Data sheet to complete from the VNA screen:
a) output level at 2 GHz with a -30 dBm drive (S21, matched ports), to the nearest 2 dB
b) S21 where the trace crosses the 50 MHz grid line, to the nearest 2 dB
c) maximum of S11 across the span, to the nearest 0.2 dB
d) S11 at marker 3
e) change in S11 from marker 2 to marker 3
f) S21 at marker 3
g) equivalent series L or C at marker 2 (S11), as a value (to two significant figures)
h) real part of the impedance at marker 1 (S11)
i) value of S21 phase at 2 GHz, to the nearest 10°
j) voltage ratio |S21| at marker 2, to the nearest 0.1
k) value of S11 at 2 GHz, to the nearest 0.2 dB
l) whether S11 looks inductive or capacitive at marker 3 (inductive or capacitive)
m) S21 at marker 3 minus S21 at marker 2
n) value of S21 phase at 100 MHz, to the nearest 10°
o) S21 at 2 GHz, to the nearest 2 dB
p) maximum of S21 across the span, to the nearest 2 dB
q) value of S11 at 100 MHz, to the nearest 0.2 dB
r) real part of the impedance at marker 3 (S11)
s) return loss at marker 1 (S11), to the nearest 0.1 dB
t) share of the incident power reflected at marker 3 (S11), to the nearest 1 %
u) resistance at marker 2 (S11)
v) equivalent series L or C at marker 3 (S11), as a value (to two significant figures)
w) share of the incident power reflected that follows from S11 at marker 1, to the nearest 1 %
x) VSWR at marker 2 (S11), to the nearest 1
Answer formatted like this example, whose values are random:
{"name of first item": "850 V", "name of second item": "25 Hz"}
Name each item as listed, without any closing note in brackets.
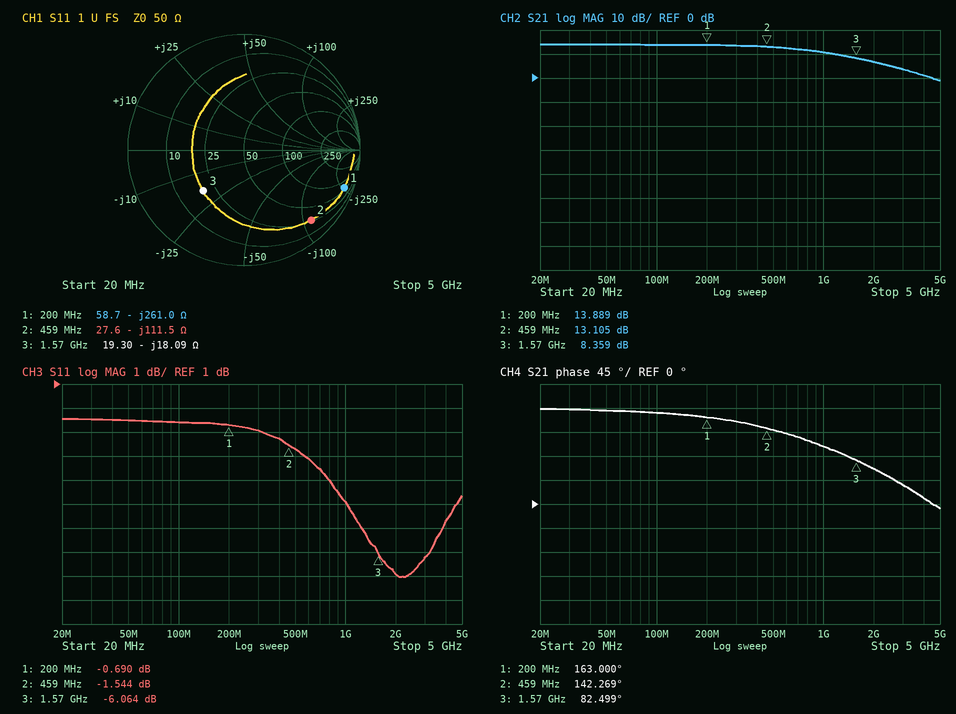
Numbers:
{"output level at 2 GHz with a -30 dBm drive (S21, matched ports), to the nearest 2 dB": "-24 dBm", "S21 where the trace crosses the 50 MHz grid line, to the nearest 2 dB": "14 dB", "maximum of S11 across the span, to the nearest 0.2 dB": "-0.4 dB", "S11 at marker 3": "-6.064 dB", "change in S11 from marker 2 to marker 3": "-4.520 dB", "S21 at marker 3": "8.359 dB", "equivalent series L or C at marker 2 (S11), as a value": "3.1 pF", "real part of the impedance at marker 1": "58.7 Ω", "value of S21 phase at 2 GHz, to the nearest 10°": "70°", "voltage ratio |S21| at marker 2, to the nearest 0.1": "4.5", "value of S11 at 2 GHz, to the nearest 0.2 dB": "-7.0 dB", "whether S11 looks inductive or capacitive at marker 3": "capacitive", "S21 at marker 3 minus S21 at marker 2": "-4.746 dB", "value of S21 phase at 100 MHz, to the nearest 10°": "170°", "S21 at 2 GHz, to the nearest 2 dB": "6 dB", "maximum of S21 across the span, to the nearest 2 dB": "14 dB", "value of S11 at 100 MHz, to the nearest 0.2 dB": "-0.6 dB", "real part of the impedance at marker 3": "19.30 Ω", "return loss at marker 1 (S11), to the nearest 0.1 dB": "0.7 dB", "share of the incident power reflected at marker 3 (S11), to the nearest 1 %": "25 %", "resistance at marker 2": "27.6 Ω", "equivalent series L or C at marker 3 (S11), as a value": "5.6 pF", "share of the incident power reflected that follows from S11 at marker 1, to the nearest 1 %": "85 %", "VSWR at marker 2 (S11), to the nearest 1": "11"}
